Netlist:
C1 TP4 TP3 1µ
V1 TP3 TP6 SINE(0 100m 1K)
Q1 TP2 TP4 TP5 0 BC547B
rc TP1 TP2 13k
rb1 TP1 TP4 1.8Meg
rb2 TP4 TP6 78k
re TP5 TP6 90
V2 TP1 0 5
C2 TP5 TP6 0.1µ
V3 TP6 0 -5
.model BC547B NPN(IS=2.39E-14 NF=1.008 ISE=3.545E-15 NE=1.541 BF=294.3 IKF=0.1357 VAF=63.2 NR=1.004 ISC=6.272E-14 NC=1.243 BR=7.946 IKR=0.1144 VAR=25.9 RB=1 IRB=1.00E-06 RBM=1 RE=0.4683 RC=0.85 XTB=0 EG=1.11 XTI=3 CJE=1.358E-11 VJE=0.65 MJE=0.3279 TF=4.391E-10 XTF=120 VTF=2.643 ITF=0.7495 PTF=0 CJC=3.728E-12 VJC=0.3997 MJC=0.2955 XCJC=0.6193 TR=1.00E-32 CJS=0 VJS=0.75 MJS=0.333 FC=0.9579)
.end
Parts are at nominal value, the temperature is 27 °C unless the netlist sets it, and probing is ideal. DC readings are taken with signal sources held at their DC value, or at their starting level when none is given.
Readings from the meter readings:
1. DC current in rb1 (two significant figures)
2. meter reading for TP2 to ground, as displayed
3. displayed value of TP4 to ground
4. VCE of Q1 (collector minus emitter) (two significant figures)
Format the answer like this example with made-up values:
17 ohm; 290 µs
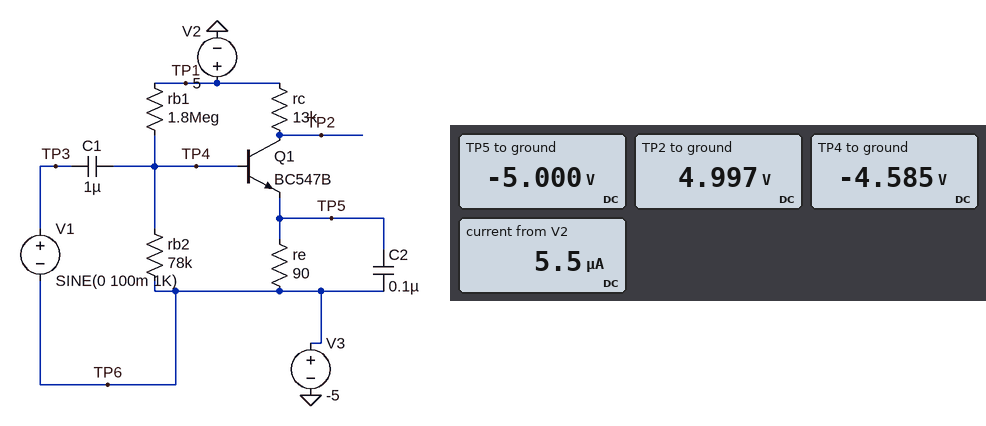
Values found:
5.3 µA; 4.997 V; -4.585 V; 10 V
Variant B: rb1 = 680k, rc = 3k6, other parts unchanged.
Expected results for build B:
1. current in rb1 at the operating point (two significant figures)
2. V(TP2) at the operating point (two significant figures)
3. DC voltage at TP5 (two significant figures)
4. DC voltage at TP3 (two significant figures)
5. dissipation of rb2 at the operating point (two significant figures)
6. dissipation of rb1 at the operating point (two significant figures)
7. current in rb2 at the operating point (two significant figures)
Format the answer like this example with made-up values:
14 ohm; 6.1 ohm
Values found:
14 µA; 650 mV; -4.9 V; -5.0 V; 7.2 µW; 130 µW; 9.6 µA
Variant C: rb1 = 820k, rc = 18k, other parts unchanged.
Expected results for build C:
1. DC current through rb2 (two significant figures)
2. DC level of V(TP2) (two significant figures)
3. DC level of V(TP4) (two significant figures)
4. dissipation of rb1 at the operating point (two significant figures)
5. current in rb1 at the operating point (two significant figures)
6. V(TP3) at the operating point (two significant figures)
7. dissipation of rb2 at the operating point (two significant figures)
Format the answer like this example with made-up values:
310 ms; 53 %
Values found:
8.6 µA; -4.8 V; -4.3 V; 110 µW; 11 µA; -5.0 V; 5.8 µW
